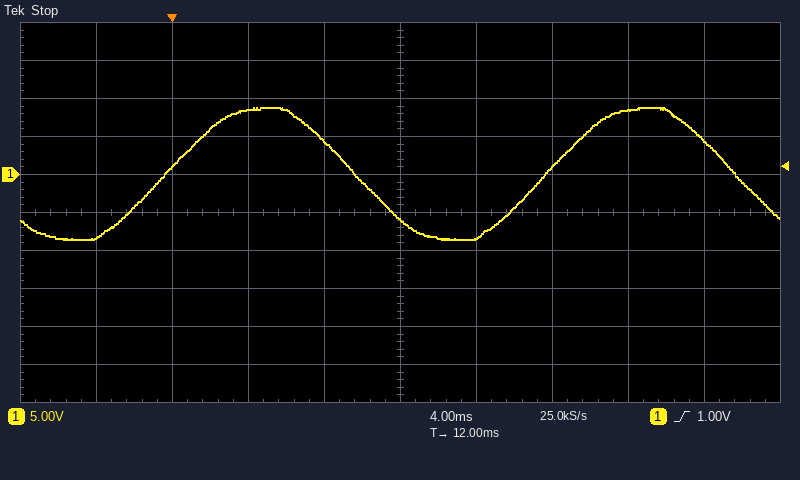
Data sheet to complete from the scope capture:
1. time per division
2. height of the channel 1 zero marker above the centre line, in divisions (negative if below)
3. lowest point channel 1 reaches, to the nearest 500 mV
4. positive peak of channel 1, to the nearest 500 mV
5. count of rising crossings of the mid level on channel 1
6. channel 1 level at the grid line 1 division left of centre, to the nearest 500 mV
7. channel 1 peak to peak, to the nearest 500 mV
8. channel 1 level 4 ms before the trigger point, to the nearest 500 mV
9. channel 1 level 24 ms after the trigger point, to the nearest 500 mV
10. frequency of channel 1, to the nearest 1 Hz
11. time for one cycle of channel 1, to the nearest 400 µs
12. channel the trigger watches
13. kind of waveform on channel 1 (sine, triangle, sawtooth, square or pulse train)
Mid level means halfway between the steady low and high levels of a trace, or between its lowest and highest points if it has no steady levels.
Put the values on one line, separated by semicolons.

4 ms; +1.0 div; -8.5 V; 9.0 V; 2; 4.5 V; 17.5 V; -8.5 V; 8.5 V; 50 Hz; 20.0 ms; channel 1; sine
